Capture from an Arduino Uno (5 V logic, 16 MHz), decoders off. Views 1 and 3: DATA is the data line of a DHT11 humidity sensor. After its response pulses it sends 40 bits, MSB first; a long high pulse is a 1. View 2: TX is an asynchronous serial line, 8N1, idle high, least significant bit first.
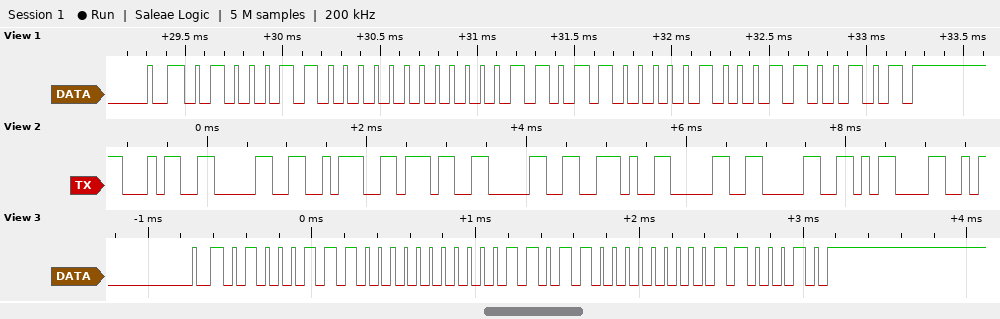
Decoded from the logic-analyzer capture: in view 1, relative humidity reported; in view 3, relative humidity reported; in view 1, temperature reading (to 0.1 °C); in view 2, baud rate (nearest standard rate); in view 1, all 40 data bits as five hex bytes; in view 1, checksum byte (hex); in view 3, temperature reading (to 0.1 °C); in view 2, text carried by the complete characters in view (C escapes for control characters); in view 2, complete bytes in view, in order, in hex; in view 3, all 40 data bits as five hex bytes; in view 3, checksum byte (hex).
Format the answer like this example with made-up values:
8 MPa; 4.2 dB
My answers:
70 %; 71 %; 27.4 °C; 9600 baud; 46 00 1B 04 65; 0x65; 27.0 °C; "40:70.00\r"; 0x34 0x30 0x3A 0x37 0x30 0x2E 0x30 0x30 0x0D; 47 00 1B 00 62; 0x62
